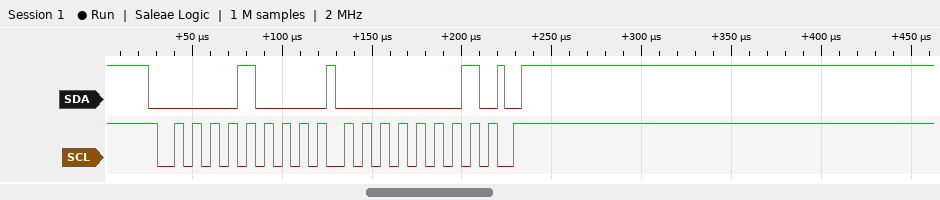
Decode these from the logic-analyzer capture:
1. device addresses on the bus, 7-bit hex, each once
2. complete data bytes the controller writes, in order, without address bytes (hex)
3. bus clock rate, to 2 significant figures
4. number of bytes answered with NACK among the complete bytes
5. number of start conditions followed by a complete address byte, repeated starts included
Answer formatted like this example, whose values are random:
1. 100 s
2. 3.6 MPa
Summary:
1. 0x04
2. 01
3. 100 kHz
4. 0
5. 1
